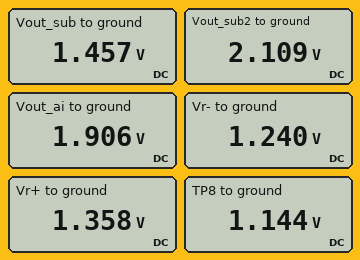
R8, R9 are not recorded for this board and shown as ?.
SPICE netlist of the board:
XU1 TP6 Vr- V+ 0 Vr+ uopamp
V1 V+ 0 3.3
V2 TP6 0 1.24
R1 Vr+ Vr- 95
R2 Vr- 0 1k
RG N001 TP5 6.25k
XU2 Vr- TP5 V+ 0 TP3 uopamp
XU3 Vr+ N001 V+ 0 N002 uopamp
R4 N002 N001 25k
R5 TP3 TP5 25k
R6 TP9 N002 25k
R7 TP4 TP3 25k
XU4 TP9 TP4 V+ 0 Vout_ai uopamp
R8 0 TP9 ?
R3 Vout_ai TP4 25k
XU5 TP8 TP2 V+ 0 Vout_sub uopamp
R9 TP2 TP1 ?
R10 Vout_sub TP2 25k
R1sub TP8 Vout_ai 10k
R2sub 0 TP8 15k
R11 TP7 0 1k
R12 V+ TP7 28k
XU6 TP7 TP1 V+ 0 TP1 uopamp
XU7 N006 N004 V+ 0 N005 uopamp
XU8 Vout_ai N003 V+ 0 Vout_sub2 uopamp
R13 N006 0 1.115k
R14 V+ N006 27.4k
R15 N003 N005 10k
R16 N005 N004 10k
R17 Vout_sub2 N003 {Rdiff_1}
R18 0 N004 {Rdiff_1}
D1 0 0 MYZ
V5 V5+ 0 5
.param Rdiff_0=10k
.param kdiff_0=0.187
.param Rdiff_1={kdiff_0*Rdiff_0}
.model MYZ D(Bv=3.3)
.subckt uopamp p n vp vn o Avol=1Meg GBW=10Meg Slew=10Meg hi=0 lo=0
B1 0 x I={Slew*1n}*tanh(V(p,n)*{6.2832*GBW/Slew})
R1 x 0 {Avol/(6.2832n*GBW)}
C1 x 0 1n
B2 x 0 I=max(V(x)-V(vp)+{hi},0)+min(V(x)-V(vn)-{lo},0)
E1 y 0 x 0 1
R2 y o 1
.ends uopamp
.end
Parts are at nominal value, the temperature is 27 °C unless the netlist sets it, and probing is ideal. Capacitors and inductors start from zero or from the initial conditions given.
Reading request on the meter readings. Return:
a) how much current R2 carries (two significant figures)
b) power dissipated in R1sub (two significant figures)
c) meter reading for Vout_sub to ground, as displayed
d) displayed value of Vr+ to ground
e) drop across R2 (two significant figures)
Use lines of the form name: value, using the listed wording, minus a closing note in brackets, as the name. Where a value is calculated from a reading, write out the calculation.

how much current R2 carries: (1.24 V) / 1 kΩ = 1.2 mA
power dissipated in R1sub: (1.906 V - 1.144 V)^2 / 10 kΩ = 58 µW
meter reading for Vout_sub to ground, as displayed: 1.457 V
displayed value of Vr+ to ground: 1.358 V
drop across R2: 1.24 V = 1.2 V
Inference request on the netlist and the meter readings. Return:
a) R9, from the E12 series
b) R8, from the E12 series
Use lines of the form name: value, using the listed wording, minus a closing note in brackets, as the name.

R9, from the E12 series: 82 kΩ
R8, from the E12 series: 68 kΩ
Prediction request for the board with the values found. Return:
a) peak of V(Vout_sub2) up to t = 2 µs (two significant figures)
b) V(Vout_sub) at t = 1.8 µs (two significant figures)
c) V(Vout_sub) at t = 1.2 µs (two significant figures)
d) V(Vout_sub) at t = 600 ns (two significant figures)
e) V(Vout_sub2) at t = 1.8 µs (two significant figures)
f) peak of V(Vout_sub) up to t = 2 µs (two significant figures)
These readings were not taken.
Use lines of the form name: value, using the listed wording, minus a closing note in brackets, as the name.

peak of V(Vout_sub2) up to t = 2 µs: 2.1 V
V(Vout_sub) at t = 1.8 µs: 1.5 V
V(Vout_sub) at t = 1.2 µs: 1.5 V
V(Vout_sub) at t = 600 ns: 1.4 V
V(Vout_sub2) at t = 1.8 µs: 2.1 V
peak of V(Vout_sub) up to t = 2 µs: 1.5 V
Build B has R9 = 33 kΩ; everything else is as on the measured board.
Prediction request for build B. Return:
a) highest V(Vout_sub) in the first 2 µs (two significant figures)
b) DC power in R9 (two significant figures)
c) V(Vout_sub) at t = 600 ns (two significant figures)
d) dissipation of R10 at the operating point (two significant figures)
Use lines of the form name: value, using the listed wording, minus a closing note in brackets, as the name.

highest V(Vout_sub) in the first 2 µs: 1.9 V
DC power in R9: 32 µW
V(Vout_sub) at t = 600 ns: 1.8 V
dissipation of R10 at the operating point: 24 µW
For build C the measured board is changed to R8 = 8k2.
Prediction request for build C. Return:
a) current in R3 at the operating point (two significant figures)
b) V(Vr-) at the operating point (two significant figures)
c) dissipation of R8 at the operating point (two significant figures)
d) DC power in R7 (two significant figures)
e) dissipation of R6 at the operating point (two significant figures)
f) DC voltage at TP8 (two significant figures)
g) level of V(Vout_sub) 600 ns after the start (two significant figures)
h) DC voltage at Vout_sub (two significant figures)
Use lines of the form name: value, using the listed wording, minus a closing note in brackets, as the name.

current in R3 at the operating point: 13 µA
V(Vr-) at the operating point: 1.2 V
dissipation of R8 at the operating point: 25 µW
DC power in R7: 4.0 µW
dissipation of R6 at the operating point: 76 µW
DC voltage at TP8: 81 mV
level of V(Vout_sub) 600 ns after the start: 35 mV
DC voltage at Vout_sub: 71 mV
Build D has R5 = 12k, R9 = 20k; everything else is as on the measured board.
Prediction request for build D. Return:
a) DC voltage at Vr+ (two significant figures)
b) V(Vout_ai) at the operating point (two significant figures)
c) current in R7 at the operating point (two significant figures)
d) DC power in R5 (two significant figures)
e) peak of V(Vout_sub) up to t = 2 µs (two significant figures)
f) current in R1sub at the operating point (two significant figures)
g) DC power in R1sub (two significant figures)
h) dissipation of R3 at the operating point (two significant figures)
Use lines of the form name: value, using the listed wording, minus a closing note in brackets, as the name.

DC voltage at Vr+: 1.4 V
V(Vout_ai) at the operating point: 1.7 V
current in R7 at the operating point: 13 µA
DC power in R5: 4.3 µW
peak of V(Vout_sub) up to t = 2 µs: 2.1 V
current in R1sub at the operating point: 66 µA
DC power in R1sub: 44 µW
dissipation of R3 at the operating point: 4.2 µW
